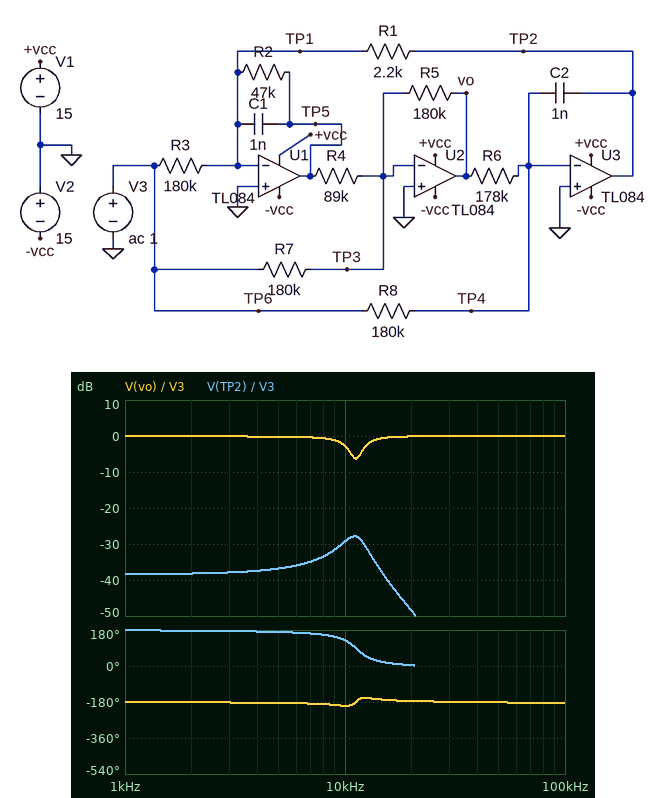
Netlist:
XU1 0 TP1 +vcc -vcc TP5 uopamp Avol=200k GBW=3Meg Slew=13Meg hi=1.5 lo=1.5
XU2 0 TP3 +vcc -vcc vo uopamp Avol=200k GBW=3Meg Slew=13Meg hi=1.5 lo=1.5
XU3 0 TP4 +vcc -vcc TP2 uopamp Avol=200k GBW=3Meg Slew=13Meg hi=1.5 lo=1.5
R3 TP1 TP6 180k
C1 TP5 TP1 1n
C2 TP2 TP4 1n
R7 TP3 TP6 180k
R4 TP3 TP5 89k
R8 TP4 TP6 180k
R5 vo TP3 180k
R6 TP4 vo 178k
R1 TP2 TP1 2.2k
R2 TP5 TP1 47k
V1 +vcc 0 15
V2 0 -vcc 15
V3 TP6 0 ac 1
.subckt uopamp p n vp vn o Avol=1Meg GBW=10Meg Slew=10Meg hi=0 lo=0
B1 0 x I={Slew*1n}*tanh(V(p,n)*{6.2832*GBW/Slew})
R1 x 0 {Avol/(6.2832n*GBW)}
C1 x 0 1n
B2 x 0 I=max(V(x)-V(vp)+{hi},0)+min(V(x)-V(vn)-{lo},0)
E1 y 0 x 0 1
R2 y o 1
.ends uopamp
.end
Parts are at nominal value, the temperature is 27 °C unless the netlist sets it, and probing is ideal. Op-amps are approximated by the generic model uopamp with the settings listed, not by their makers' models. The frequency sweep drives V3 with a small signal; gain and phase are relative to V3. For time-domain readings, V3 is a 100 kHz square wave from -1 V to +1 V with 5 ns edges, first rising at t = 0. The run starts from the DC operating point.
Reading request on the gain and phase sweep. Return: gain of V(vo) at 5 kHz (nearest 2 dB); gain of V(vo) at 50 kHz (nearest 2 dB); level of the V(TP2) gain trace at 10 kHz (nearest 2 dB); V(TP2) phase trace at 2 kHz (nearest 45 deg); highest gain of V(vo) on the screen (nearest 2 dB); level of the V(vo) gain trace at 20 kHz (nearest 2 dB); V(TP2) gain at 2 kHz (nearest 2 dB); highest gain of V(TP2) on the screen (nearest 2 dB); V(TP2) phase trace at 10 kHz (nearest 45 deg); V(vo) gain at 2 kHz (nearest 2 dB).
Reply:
0 dB
0 dB
-30 dB
180 deg
0 dB
0 dB
-38 dB
-28 dB
135 deg
0 dB
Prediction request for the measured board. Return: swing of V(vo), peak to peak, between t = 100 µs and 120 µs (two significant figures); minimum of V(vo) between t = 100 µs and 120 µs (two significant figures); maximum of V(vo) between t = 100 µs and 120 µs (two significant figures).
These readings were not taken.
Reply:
2.0 V
-970 mV
1.1 V
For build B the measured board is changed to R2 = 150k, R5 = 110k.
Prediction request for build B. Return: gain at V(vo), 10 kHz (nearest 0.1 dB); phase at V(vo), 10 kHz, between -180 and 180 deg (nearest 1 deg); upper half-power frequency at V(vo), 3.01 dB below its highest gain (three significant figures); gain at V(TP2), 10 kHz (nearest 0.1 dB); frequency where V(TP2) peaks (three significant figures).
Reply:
-3.1 dB
5 deg
9.13 kHz
-16.4 dB
8.83 kHz
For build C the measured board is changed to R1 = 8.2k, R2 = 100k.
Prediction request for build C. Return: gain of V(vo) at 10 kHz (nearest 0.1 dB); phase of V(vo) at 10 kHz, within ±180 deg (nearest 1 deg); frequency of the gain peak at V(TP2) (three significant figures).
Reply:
-0.2 dB
-166 deg
5.80 kHz
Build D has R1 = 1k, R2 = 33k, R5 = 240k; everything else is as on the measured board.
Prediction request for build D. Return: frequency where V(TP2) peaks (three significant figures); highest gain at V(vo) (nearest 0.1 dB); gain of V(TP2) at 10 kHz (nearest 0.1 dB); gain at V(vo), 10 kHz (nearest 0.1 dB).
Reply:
19.1 kHz
7.1 dB
-38.8 dB
-1.3 dB
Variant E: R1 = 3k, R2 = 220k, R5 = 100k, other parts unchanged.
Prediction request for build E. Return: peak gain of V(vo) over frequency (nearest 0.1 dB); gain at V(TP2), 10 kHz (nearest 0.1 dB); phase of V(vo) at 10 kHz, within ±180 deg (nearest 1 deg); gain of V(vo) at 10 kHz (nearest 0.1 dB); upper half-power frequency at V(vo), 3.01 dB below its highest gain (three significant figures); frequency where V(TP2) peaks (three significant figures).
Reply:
14.2 dB
-21.6 dB
-115 deg
-16.4 dB
7.47 kHz
7.23 kHz
